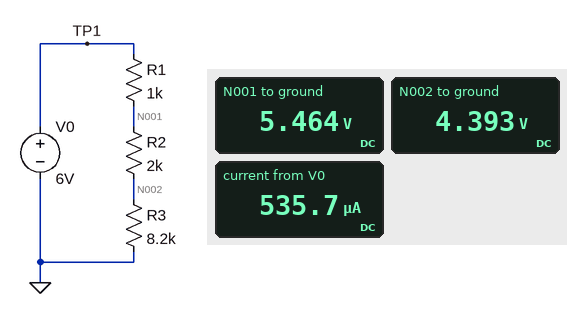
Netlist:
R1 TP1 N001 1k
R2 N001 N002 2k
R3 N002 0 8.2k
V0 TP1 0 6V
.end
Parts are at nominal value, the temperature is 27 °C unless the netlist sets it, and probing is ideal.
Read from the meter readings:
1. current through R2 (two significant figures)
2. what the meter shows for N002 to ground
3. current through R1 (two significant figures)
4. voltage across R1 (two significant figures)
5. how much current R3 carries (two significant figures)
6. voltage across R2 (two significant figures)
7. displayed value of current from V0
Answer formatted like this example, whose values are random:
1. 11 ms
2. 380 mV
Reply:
1. 540 µA
2. 4.393 V
3. 540 µA
4. 540 mV
5. 540 µA
6. 1.1 V
7. 535.7 µA
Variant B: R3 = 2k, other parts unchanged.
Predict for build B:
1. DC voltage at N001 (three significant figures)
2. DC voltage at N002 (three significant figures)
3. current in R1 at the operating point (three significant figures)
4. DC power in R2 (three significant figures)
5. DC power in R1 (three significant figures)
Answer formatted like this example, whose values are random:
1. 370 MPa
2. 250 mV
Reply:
1. 4.80 V
2. 2.40 V
3. 1.20 mA
4. 2.88 mW
5. 1.44 mW
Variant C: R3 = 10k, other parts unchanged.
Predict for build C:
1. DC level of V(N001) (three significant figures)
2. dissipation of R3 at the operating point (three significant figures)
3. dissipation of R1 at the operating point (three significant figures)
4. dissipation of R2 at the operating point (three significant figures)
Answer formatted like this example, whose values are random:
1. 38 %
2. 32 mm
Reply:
1. 5.54 V
2. 2.13 mW
3. 213 µW
4. 426 µW
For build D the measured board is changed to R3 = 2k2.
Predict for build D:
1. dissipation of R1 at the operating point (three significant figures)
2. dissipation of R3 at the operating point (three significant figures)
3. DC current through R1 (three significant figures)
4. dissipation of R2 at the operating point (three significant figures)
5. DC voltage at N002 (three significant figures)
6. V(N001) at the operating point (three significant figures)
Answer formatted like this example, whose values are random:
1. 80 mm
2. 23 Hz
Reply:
1. 1.33 mW
2. 2.93 mW
3. 1.15 mA
4. 2.66 mW
5. 2.54 V
6. 4.85 V
